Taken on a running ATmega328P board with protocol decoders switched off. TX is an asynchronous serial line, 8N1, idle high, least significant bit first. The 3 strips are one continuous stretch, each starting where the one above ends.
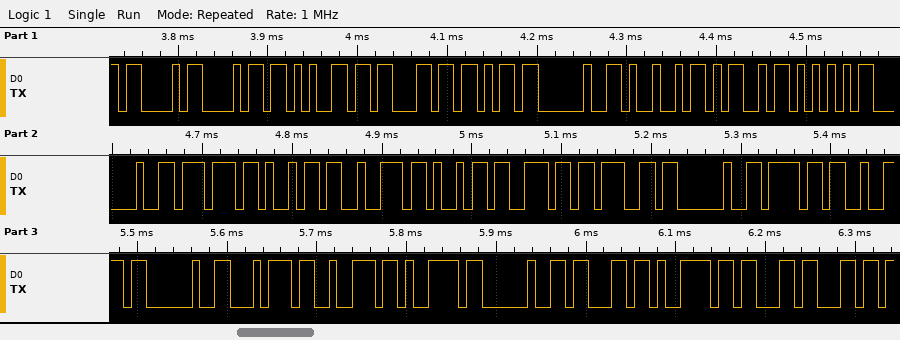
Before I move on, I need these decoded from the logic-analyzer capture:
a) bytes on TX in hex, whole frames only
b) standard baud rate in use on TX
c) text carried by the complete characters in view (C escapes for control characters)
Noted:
43 68 65 63 6B 20 49 4D 55 20 77 69 72 69 6E 67 20 6F 72 20 74 72 79 20 63 79 63 6C
115200 baud
"Check IMU wiring or try cycl"
